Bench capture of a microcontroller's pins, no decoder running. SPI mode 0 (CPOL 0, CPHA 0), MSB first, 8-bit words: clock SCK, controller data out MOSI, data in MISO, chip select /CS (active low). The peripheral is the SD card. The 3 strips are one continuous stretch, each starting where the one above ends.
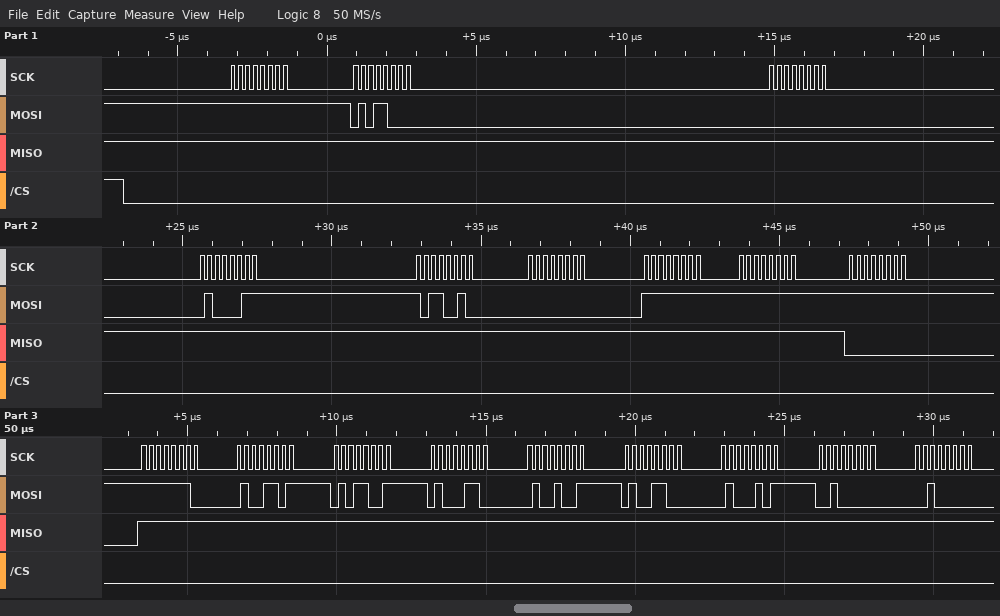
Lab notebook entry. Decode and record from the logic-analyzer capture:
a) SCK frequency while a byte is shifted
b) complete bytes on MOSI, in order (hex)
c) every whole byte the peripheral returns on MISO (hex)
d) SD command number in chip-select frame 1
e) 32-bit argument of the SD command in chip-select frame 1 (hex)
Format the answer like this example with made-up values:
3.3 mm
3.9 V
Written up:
4 MHz
FF 58 00 43 B2 00 FF FF FF FE 4D 59 46 49 4C 45 20 20
FF FF FF FF FF FF FF FF 00 FF FF FF FF FF FF FF FF FF
CMD24
0x0043B200
